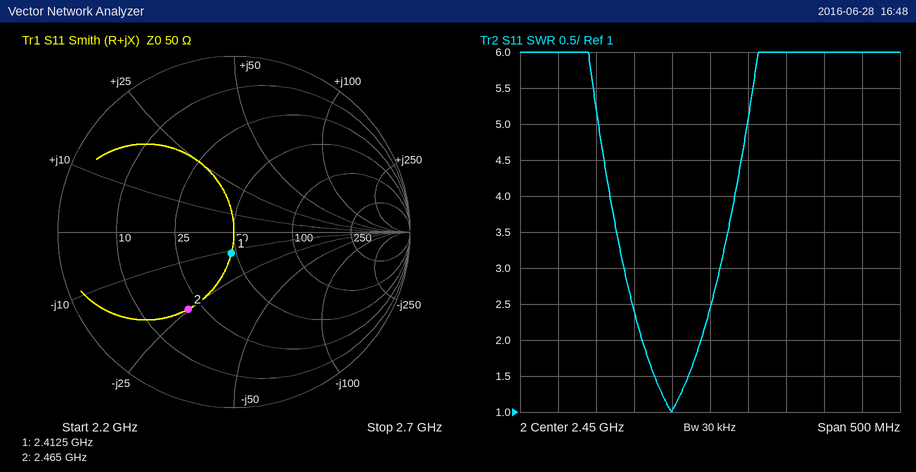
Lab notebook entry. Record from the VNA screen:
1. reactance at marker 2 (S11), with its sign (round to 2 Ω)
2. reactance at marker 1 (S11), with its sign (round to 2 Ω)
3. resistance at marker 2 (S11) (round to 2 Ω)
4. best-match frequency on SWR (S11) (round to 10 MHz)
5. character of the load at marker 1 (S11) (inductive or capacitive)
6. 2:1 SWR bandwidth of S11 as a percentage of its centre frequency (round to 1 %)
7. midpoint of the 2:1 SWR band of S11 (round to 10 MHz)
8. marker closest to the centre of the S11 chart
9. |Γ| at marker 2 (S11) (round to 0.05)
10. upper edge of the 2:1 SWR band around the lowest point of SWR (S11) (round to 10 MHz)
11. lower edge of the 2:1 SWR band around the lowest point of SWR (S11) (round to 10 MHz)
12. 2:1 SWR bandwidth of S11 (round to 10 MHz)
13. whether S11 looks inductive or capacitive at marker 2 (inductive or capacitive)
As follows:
-24 Ω
-12 Ω
20 Ω
2.40 GHz
capacitive
3 %
2.40 GHz
marker 1
0.50
2.44 GHz
2.36 GHz
80 MHz
capacitive
